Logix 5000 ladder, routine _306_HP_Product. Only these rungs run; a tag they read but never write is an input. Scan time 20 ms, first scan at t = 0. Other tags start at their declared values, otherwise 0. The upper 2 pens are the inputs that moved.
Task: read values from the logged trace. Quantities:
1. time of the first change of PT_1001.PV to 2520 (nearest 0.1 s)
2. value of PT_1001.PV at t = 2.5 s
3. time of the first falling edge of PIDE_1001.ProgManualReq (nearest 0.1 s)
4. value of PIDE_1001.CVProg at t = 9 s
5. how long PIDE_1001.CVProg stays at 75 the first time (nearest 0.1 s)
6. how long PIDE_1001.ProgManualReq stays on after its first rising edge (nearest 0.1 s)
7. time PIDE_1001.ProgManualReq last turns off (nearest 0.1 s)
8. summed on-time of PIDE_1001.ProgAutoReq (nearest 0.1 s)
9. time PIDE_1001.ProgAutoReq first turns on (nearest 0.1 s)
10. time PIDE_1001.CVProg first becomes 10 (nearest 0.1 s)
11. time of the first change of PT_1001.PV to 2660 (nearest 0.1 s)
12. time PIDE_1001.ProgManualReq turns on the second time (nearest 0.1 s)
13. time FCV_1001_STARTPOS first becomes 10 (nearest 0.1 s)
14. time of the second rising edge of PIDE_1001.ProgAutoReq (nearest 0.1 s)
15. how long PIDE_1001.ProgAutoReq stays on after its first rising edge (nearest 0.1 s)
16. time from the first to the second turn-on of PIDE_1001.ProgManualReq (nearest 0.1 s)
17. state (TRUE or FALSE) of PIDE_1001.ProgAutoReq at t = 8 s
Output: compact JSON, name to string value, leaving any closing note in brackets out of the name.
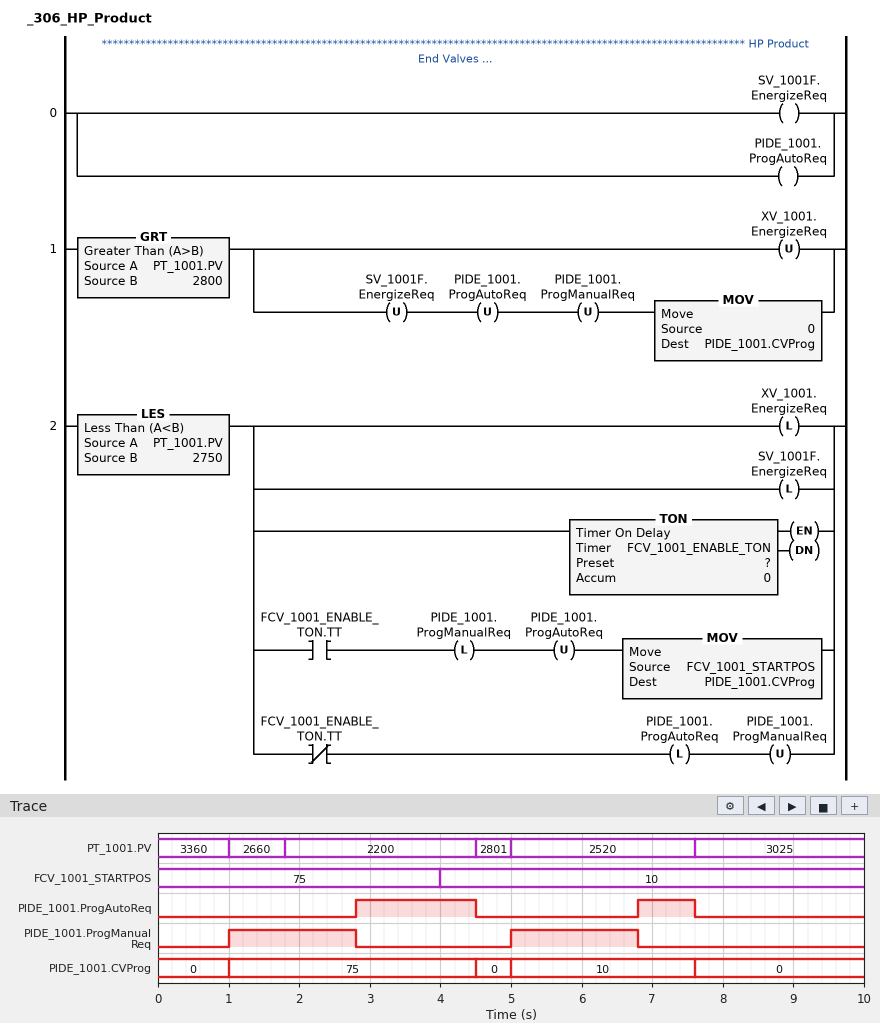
{"time of the first change of PT_1001.PV to 2520": "5.0 s", "value of PT_1001.PV at t = 2.5 s": "2200", "time of the first falling edge of PIDE_1001.ProgManualReq": "2.8 s", "value of PIDE_1001.CVProg at t = 9 s": "0", "how long PIDE_1001.CVProg stays at 75 the first time": "3.5 s", "how long PIDE_1001.ProgManualReq stays on after its first rising edge": "1.8 s", "time PIDE_1001.ProgManualReq last turns off": "6.8 s", "summed on-time of PIDE_1001.ProgAutoReq": "2.5 s", "time PIDE_1001.ProgAutoReq first turns on": "2.8 s", "time PIDE_1001.CVProg first becomes 10": "5.0 s", "time of the first change of PT_1001.PV to 2660": "1.0 s", "time PIDE_1001.ProgManualReq turns on the second time": "5.0 s", "time FCV_1001_STARTPOS first becomes 10": "4.0 s", "time of the second rising edge of PIDE_1001.ProgAutoReq": "6.8 s", "how long PIDE_1001.ProgAutoReq stays on after its first rising edge": "1.7 s", "time from the first to the second turn-on of PIDE_1001.ProgManualReq": "4.0 s", "state (TRUE or FALSE) of PIDE_1001.ProgAutoReq at t = 8 s": "FALSE"}
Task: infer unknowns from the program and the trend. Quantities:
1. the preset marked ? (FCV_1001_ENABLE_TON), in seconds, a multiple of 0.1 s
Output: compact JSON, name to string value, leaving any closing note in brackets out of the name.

{"the preset marked ? (FCV_1001_ENABLE_TON), in seconds, a multiple of 0.1 s": "1.8 s"}
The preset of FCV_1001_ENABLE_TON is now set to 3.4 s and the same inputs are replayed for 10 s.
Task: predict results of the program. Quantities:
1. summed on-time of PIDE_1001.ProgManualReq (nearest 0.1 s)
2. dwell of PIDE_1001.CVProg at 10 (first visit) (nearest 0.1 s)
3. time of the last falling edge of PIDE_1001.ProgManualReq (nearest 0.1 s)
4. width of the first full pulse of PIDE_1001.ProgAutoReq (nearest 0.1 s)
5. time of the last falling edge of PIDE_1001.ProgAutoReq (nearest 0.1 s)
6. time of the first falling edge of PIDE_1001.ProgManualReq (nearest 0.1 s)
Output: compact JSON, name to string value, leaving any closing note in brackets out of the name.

{"summed on-time of PIDE_1001.ProgManualReq": "6.0 s", "dwell of PIDE_1001.CVProg at 10 (first visit)": "0.5 s", "time of the last falling edge of PIDE_1001.ProgManualReq": "7.6 s", "width of the first full pulse of PIDE_1001.ProgAutoReq": "0.1 s", "time of the last falling edge of PIDE_1001.ProgAutoReq": "4.5 s", "time of the first falling edge of PIDE_1001.ProgManualReq": "4.4 s"}
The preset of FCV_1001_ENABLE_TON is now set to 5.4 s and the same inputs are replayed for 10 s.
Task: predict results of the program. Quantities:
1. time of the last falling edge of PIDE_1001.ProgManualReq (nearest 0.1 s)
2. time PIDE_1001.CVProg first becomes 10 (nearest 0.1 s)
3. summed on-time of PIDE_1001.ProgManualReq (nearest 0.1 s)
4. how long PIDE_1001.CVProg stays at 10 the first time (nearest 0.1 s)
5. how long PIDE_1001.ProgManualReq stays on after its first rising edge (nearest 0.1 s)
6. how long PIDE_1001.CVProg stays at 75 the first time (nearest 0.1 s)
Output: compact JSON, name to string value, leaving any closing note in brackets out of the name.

{"time of the last falling edge of PIDE_1001.ProgManualReq": "7.6 s", "time PIDE_1001.CVProg first becomes 10": "4.0 s", "summed on-time of PIDE_1001.ProgManualReq": "6.1 s", "how long PIDE_1001.CVProg stays at 10 the first time": "0.5 s", "how long PIDE_1001.ProgManualReq stays on after its first rising edge": "3.5 s", "how long PIDE_1001.CVProg stays at 75 the first time": "3.0 s"}
